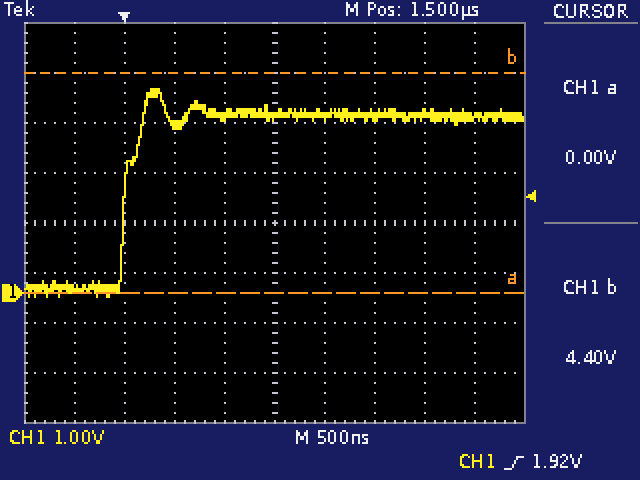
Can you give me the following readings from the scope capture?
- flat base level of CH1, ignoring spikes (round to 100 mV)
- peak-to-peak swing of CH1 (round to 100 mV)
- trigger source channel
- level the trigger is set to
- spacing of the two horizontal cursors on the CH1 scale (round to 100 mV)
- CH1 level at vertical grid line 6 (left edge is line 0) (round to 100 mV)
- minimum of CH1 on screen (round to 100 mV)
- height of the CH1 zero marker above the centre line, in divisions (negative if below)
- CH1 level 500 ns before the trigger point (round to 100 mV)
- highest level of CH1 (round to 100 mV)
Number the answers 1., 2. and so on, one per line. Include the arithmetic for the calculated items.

1. 100 mV
2. 4.1 V − (-100 mV) = 4.2 V
3. CH1
4. 1.92 V
5. 4.4 V
6. 3.5 V
7. -100 mV
8. -1.4 div
9. 100 mV
10. 4.1 V
